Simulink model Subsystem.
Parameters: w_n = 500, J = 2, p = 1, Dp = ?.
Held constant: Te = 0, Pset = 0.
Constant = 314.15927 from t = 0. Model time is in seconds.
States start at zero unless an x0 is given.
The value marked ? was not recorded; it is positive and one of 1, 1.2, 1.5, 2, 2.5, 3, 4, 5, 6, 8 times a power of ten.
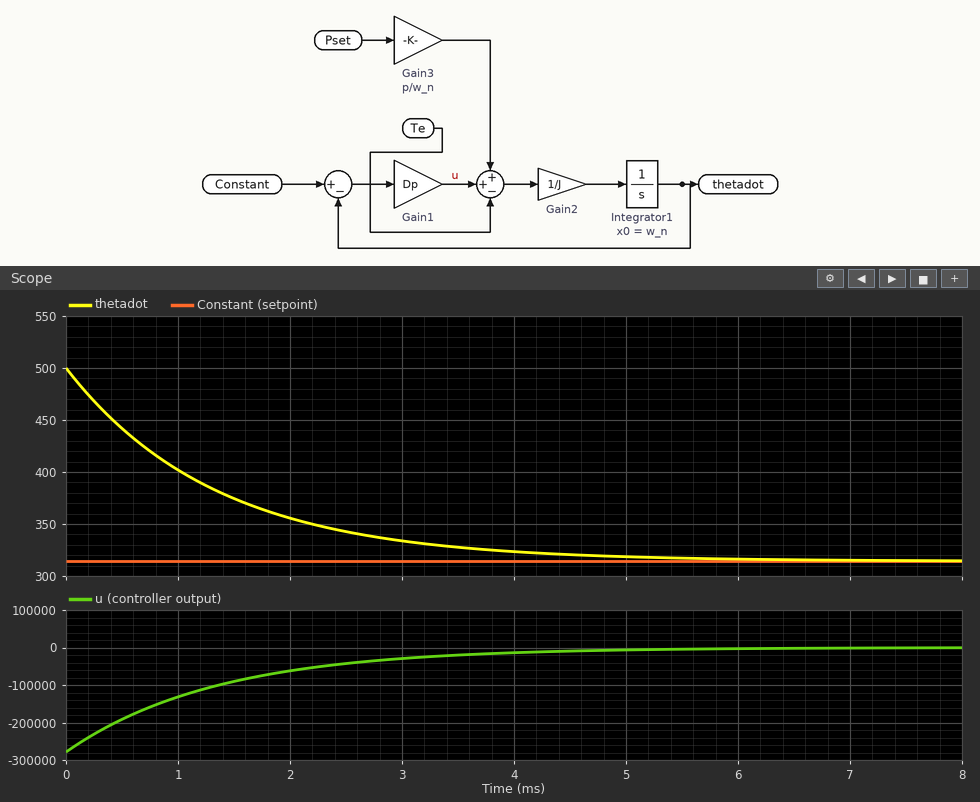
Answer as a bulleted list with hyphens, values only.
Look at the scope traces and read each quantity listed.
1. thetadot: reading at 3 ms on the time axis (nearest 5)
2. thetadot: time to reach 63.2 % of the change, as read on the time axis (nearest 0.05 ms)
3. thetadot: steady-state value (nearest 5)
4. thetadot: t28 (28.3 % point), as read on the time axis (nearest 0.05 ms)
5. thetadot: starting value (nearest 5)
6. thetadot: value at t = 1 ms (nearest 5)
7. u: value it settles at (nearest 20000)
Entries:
- 335
- 1.35 ms
- 315
- 0.45 ms
- 500
- 400
- 0
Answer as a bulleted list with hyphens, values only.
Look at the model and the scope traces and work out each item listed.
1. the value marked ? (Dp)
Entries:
- 1500
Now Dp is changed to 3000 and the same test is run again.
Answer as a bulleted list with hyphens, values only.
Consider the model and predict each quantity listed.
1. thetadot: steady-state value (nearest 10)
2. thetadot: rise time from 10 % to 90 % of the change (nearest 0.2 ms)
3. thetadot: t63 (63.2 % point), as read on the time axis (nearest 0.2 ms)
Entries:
- 310
- 1.4 ms
- 0.6 ms
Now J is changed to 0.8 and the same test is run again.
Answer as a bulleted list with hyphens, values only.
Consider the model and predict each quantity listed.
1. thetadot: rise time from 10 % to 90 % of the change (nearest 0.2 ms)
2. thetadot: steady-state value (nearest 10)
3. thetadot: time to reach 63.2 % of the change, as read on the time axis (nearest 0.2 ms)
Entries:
- 1.2 ms
- 310
- 0.6 ms
